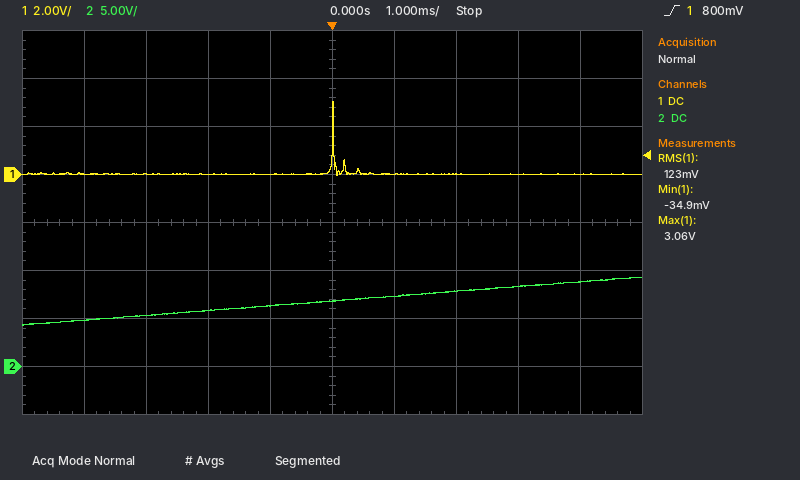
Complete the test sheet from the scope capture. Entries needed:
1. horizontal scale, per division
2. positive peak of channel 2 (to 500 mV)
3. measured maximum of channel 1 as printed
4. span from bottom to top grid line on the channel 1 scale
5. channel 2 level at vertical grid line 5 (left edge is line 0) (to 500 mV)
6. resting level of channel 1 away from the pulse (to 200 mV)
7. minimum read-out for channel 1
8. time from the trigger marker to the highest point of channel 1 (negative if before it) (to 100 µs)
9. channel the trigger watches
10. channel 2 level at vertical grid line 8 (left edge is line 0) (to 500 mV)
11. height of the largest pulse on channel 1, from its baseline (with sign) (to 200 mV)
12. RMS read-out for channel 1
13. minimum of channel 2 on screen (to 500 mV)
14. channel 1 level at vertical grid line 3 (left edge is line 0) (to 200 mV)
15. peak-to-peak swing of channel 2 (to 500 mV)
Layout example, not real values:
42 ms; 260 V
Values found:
1 ms; 9.5 V; 3.06 V; 16 V; 7.0 V; 0.0 V; -34.9 mV; 0.0 ms; channel 1; 8.5 V; +3.0 V; 123 mV; 4.5 V; 0.0 V; 5.0 V
